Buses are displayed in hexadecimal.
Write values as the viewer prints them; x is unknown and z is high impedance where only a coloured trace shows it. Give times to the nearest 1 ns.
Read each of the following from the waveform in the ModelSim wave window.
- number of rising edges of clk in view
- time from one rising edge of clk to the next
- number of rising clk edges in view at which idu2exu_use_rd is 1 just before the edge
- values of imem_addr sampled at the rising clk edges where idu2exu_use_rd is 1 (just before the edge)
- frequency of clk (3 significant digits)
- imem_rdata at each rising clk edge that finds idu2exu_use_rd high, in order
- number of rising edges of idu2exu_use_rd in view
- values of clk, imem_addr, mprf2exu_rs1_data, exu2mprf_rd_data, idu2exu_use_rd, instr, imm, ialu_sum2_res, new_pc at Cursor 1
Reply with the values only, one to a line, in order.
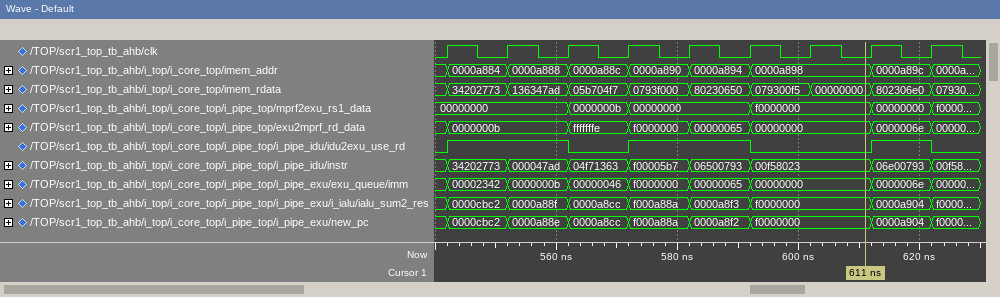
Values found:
9
10 ns
5
0000a884, 0000a888, 0000a890, 0000a894, 0000a89c
100 MHz
34202773, 136347ad, 0793f000, 80230650, 802306e0
3
clk=0, imem_addr=0000a898, mprf2exu_rs1_data=f0000000, exu2mprf_rd_data=00000000, idu2exu_use_rd=0, instr=00f58023, imm=00000000, ialu_sum2_res=f0000000, new_pc=f0000000
